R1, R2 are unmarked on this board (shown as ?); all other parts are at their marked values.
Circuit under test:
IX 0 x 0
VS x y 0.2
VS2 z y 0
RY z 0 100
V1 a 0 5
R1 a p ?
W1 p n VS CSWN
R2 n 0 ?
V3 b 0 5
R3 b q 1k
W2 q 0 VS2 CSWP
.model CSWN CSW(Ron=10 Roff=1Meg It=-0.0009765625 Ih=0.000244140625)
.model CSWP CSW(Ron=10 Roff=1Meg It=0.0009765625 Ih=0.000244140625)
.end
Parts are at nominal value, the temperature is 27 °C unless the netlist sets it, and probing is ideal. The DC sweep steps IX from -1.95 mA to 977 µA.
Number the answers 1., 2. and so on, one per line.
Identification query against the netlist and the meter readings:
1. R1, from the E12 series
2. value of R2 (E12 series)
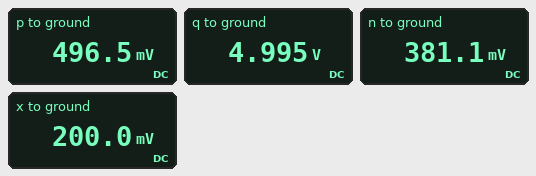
1. 390 Ω
2. 33 Ω
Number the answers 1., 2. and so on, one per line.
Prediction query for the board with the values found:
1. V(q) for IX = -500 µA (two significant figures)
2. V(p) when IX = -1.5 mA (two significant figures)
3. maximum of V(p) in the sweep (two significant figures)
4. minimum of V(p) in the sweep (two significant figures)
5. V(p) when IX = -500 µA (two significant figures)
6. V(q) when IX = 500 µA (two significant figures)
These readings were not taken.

1. 5.0 V
2. 5.0 V
3. 5.0 V
4. 500 mV
5. 500 mV
6. 5.0 V
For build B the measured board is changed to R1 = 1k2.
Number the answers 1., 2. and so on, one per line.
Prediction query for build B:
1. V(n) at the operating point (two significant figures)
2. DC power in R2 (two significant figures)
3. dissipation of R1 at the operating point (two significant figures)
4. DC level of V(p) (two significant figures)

1. 130 mV
2. 530 µW
3. 19 mW
4. 170 mV
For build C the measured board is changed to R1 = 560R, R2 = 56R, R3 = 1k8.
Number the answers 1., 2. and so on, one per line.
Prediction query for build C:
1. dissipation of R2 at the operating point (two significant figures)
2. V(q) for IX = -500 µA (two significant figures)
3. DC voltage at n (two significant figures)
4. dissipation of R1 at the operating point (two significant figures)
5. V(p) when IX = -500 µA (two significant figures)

1. 3.6 mW
2. 5.0 V
3. 450 mV
4. 36 mW
5. 530 mV
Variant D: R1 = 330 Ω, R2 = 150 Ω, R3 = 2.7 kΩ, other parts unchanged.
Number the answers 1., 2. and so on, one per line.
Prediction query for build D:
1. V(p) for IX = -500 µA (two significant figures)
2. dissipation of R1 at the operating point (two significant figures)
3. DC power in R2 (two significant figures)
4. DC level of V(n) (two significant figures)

1. 1.6 V
2. 34 mW
3. 16 mW
4. 1.5 V
